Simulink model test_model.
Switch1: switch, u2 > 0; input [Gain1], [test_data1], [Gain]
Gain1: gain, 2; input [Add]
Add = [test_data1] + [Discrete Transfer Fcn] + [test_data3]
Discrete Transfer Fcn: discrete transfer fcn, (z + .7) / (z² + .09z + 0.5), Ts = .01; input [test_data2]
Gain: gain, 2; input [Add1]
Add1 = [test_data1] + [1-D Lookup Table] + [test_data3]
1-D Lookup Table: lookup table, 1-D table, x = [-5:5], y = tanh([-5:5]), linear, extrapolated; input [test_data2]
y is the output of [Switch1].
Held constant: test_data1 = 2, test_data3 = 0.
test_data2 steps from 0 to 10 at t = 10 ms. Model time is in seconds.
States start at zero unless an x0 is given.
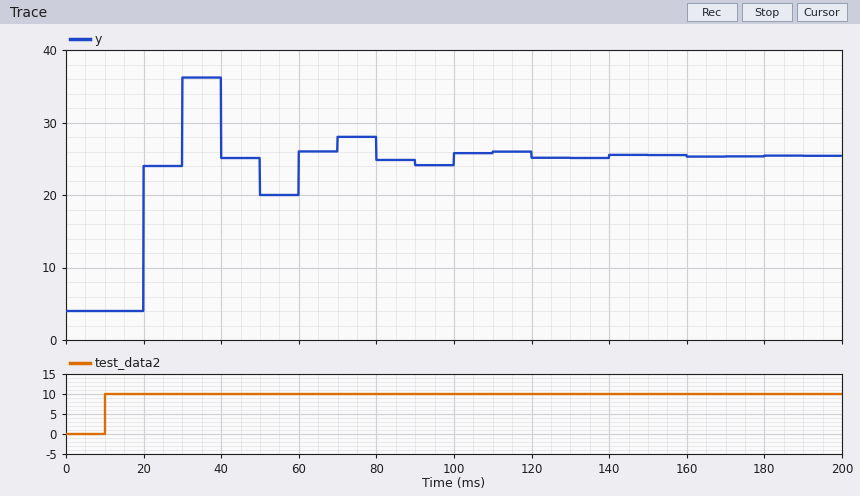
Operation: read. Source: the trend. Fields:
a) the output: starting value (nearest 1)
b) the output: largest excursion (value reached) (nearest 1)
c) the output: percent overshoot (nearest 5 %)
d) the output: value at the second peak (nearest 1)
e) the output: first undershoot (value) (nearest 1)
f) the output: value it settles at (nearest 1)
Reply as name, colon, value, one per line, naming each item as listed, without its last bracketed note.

the output: starting value: 4
the output: largest excursion (value reached): 36
the output: percent overshoot: 50 %
the output: value at the second peak: 28
the output: first undershoot (value): 20
the output: value it settles at: 25
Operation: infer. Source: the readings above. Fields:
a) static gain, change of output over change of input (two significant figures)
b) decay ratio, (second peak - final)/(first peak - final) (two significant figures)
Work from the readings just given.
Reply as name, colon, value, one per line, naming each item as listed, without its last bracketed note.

static gain, change of output over change of input: 2.1
decay ratio, (second peak - final)/(first peak - final): 0.27
